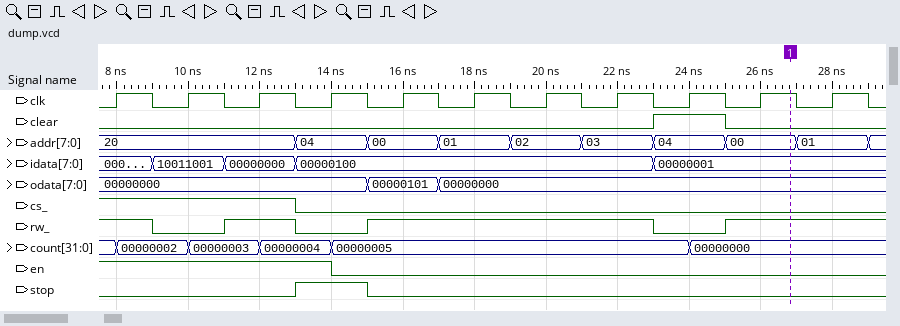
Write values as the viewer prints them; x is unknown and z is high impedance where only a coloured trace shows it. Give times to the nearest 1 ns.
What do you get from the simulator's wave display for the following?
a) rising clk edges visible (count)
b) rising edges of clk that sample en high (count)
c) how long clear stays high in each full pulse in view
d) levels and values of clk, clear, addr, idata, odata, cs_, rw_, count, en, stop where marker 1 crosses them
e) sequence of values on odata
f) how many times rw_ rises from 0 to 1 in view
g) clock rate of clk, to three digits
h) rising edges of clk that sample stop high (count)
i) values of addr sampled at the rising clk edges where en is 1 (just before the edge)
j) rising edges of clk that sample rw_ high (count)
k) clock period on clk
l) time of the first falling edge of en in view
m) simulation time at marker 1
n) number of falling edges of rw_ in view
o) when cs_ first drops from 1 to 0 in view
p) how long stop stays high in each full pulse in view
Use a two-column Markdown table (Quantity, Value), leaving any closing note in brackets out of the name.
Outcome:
| Quantity | Value |
|---|---|
| rising clk edges visible | 11 |
| rising edges of clk that sample en high | 4 |
| how long clear stays high in each full pulse in view | 2 ns |
| levels and values of clk, clear, addr, idata, odata, cs_, rw_, count, en, stop where marker 1 crosses them | clk=1, clear=0, addr=00, idata=00000001, odata=00000000, cs_=0, rw_=1, count=00000000, en=0, stop=0 |
| sequence of values on odata | 00000000, 00000101, 00000000 |
| how many times rw_ rises from 0 to 1 in view | 3 |
| clock rate of clk, to three digits | 500 MHz |
| rising edges of clk that sample stop high | 1 |
| values of addr sampled at the rising clk edges where en is 1 | 20, 20, 20, 04 |
| rising edges of clk that sample rw_ high | 8 |
| clock period on clk | 2 ns |
| time of the first falling edge of en in view | 14 ns |
| simulation time at marker 1 | 27 ns |
| number of falling edges of rw_ in view | 3 |
| when cs_ first drops from 1 to 0 in view | 13 ns |
| how long stop stays high in each full pulse in view | 2 ns |
